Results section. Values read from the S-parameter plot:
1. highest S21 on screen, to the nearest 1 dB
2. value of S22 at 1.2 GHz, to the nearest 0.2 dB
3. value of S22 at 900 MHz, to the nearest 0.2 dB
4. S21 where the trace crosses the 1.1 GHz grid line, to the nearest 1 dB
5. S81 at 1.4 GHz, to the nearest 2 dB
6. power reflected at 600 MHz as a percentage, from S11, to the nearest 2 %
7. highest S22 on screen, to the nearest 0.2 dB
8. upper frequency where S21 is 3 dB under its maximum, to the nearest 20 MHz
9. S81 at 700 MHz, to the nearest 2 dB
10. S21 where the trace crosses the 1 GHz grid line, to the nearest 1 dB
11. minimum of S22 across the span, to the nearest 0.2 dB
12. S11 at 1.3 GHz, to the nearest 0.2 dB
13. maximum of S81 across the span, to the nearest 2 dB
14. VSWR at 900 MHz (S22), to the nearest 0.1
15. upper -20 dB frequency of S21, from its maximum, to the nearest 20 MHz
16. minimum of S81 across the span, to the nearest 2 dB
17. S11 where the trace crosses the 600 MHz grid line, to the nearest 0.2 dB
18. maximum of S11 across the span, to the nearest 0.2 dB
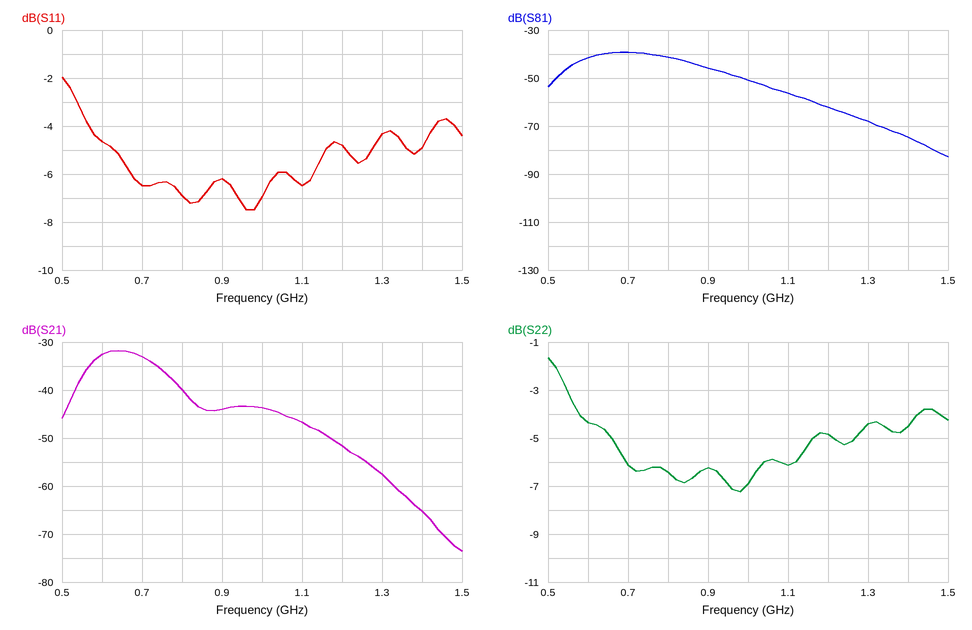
-32 dB
-4.8 dB
-6.2 dB
-47 dB
-74 dB
34 %
-1.6 dB
740 MHz
-40 dB
-44 dB
-7.2 dB
-4.4 dB
-40 dB
2.9
1.20 GHz
-82 dB
-4.6 dB
-2.0 dB
